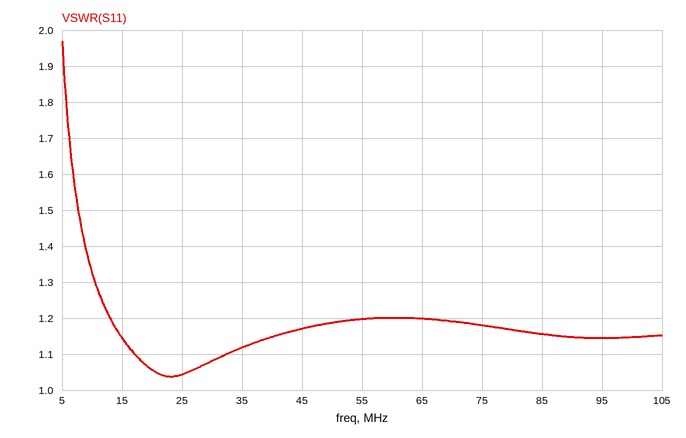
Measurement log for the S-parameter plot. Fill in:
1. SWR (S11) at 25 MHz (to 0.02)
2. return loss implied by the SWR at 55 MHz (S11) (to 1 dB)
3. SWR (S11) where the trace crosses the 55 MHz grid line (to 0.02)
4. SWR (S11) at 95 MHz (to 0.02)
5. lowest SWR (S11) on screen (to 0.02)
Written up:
1.04
21 dB
1.20
1.14
1.04
